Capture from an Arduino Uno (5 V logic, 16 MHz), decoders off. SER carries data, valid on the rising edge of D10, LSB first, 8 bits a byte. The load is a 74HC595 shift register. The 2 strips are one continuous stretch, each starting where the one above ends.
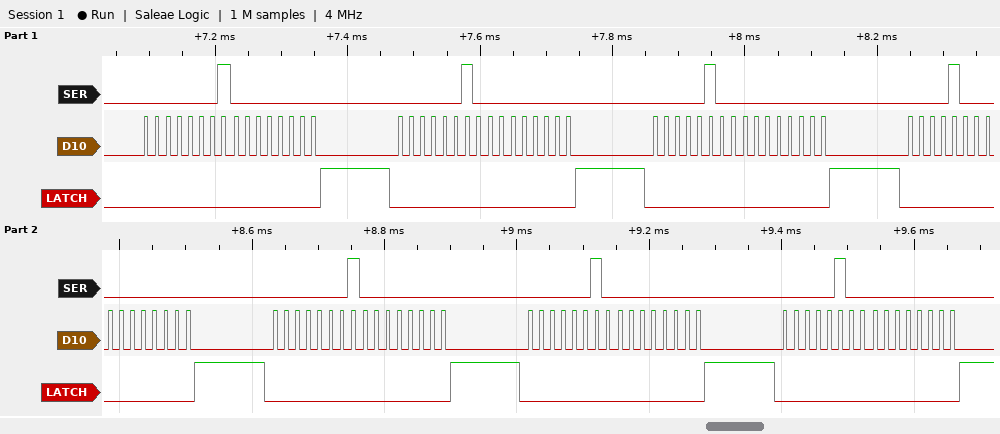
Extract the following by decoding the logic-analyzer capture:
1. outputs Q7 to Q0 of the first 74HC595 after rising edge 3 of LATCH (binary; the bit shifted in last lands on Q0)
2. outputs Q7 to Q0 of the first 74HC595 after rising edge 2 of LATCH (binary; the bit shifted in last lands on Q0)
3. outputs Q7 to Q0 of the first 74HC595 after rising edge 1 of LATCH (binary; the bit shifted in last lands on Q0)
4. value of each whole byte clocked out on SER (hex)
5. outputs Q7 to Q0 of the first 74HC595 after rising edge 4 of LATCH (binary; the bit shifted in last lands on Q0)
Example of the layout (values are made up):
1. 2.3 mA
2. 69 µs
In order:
1. 00000000
2. 00000000
3. 00000000
4. 0x80 0x00 0x40 0x00 0x20 0x00 0x10 0x00 0x80 0x00 0x40 0x00 0x20 0x00
5. 00000000
